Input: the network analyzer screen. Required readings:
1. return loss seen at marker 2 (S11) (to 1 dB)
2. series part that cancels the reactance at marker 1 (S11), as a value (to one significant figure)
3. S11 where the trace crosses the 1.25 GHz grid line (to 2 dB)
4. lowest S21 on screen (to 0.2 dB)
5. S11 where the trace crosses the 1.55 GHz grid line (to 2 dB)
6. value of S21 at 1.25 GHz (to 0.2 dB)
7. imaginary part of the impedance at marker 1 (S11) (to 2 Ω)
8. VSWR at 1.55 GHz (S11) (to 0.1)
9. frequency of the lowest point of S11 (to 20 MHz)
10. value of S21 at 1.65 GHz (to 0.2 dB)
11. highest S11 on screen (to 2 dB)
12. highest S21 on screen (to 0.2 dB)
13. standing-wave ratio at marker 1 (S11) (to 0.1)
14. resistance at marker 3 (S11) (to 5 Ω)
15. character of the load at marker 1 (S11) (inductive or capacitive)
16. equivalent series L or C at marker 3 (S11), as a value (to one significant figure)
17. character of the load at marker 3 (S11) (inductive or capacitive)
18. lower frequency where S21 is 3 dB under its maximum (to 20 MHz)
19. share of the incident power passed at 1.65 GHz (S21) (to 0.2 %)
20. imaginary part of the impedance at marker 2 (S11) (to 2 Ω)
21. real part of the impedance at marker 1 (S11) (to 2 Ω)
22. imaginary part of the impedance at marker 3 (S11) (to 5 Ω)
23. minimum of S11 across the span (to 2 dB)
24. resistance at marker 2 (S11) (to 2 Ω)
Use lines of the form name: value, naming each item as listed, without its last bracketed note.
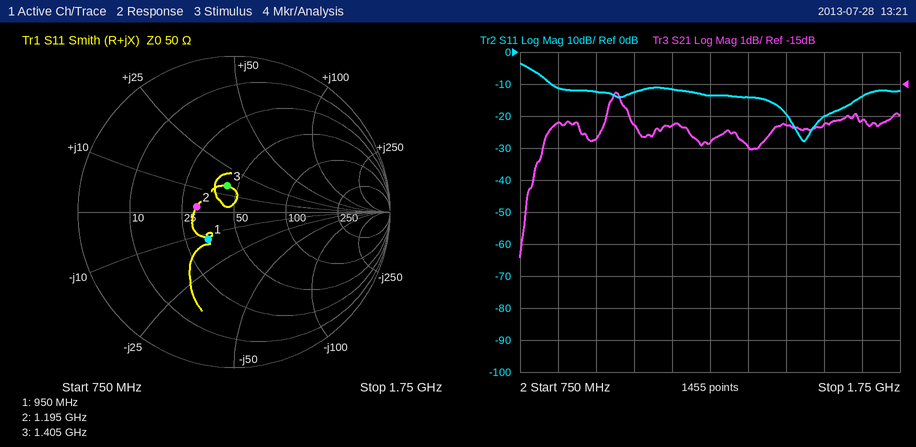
return loss seen at marker 2 (S11): 12 dB
series part that cancels the reactance at marker 1 (S11), as a value: 2 nH
S11 where the trace crosses the 1.25 GHz grid line: -14 dB
lowest S21 on screen: -20.4 dB
S11 where the trace crosses the 1.55 GHz grid line: -20 dB
value of S21 at 1.25 GHz: -16.8 dB
imaginary part of the impedance at marker 1 (S11): -12 Ω
VSWR at 1.55 GHz (S11): 1.2
frequency of the lowest point of S11: 1.50 GHz
value of S21 at 1.65 GHz: -16.2 dB
highest S11 on screen: -4 dB
highest S21 on screen: -15.2 dB
standing-wave ratio at marker 1 (S11): 1.6
resistance at marker 3 (S11): 45 Ω
character of the load at marker 1 (S11): capacitive
equivalent series L or C at marker 3 (S11), as a value: 2 nH
character of the load at marker 3 (S11): inductive
lower frequency where S21 is 3 dB under its maximum: 780 MHz
share of the incident power passed at 1.65 GHz (S21): 2.4 %
imaginary part of the impedance at marker 2 (S11): +2 Ω
real part of the impedance at marker 1 (S11): 34 Ω
imaginary part of the impedance at marker 3 (S11): +15 Ω
minimum of S11 across the span: -28 dB
resistance at marker 2 (S11): 30 Ω
